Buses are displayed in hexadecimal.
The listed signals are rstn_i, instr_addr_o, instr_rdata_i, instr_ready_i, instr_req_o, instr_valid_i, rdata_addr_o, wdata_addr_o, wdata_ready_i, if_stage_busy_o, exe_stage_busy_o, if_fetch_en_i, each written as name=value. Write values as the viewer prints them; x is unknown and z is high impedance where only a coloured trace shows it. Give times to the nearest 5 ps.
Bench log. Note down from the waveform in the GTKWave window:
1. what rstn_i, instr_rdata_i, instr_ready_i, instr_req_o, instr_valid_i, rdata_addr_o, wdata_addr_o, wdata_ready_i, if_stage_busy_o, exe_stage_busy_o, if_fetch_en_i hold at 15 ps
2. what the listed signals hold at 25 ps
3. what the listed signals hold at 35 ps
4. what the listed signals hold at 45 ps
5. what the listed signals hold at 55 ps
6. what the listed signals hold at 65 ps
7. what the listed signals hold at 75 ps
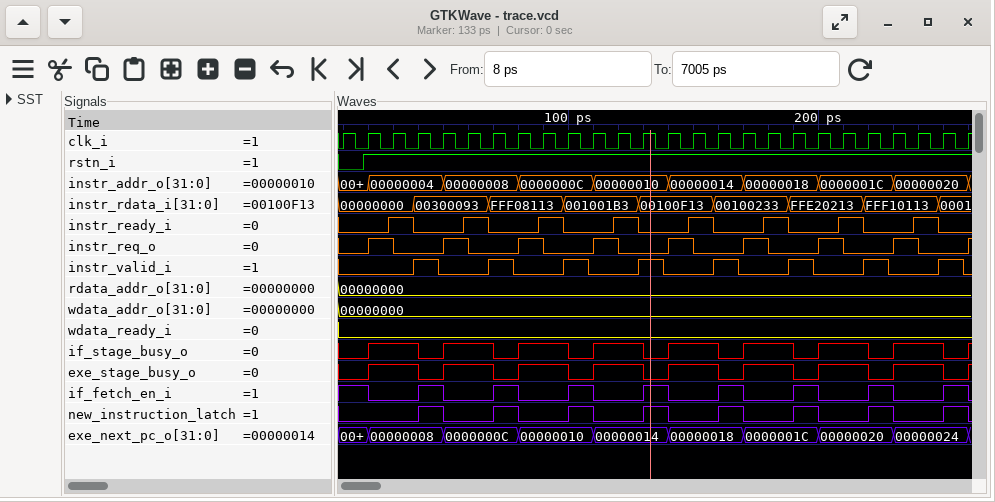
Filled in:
rstn_i=0, instr_rdata_i=00000000, instr_ready_i=0, instr_req_o=0, instr_valid_i=0, rdata_addr_o=00000000, wdata_addr_o=00000000, wdata_ready_i=0, if_stage_busy_o=0, exe_stage_busy_o=0, if_fetch_en_i=1
rstn_i=1, instr_addr_o=00000004, instr_rdata_i=00000000, instr_ready_i=0, instr_req_o=1, instr_valid_i=0, rdata_addr_o=00000000, wdata_addr_o=00000000, wdata_ready_i=0, if_stage_busy_o=1, exe_stage_busy_o=1, if_fetch_en_i=0
rstn_i=1, instr_addr_o=00000004, instr_rdata_i=00000000, instr_ready_i=1, instr_req_o=0, instr_valid_i=0, rdata_addr_o=00000000, wdata_addr_o=00000000, wdata_ready_i=0, if_stage_busy_o=1, exe_stage_busy_o=1, if_fetch_en_i=0
rstn_i=1, instr_addr_o=00000004, instr_rdata_i=00300093, instr_ready_i=0, instr_req_o=0, instr_valid_i=1, rdata_addr_o=00000000, wdata_addr_o=00000000, wdata_ready_i=0, if_stage_busy_o=0, exe_stage_busy_o=0, if_fetch_en_i=1
rstn_i=1, instr_addr_o=00000008, instr_rdata_i=00300093, instr_ready_i=0, instr_req_o=1, instr_valid_i=0, rdata_addr_o=00000000, wdata_addr_o=00000000, wdata_ready_i=0, if_stage_busy_o=1, exe_stage_busy_o=1, if_fetch_en_i=0
rstn_i=1, instr_addr_o=00000008, instr_rdata_i=00300093, instr_ready_i=1, instr_req_o=0, instr_valid_i=0, rdata_addr_o=00000000, wdata_addr_o=00000000, wdata_ready_i=0, if_stage_busy_o=1, exe_stage_busy_o=1, if_fetch_en_i=0
rstn_i=1, instr_addr_o=00000008, instr_rdata_i=FFF08113, instr_ready_i=0, instr_req_o=0, instr_valid_i=1, rdata_addr_o=00000000, wdata_addr_o=00000000, wdata_ready_i=0, if_stage_busy_o=0, exe_stage_busy_o=0, if_fetch_en_i=1
